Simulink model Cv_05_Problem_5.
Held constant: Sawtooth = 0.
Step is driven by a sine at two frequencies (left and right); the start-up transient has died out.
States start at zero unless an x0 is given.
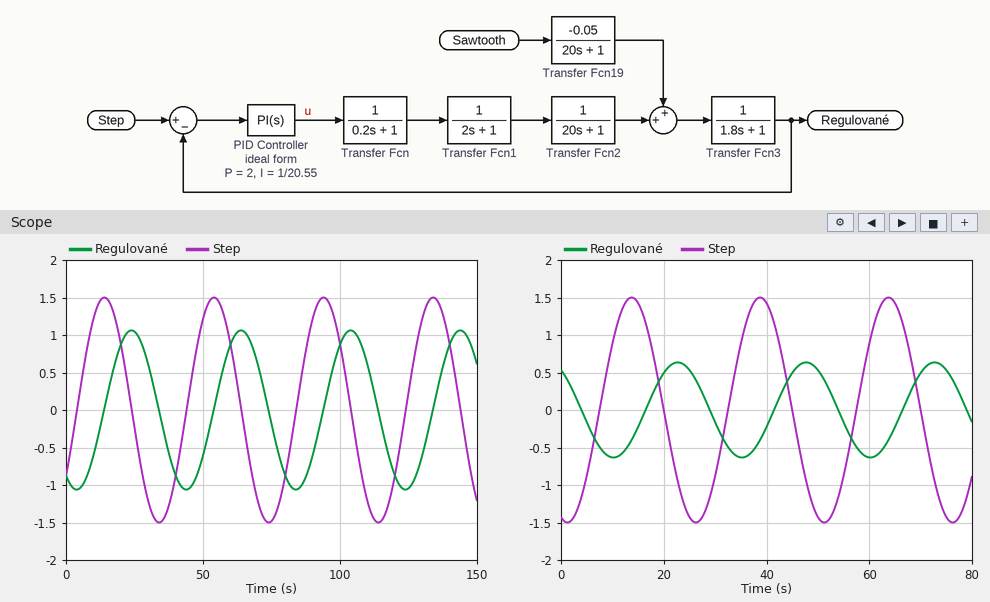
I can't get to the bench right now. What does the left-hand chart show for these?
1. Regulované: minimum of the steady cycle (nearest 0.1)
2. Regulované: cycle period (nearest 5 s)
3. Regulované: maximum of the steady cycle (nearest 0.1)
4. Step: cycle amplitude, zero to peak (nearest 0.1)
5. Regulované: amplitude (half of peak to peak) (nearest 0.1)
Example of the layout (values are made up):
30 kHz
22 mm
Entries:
-1.1
40 s
1.1
1.5
1.1
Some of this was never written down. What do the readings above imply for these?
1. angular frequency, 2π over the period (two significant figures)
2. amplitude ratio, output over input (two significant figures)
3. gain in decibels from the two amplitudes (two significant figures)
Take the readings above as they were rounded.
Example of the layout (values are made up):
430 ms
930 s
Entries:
0.16 rad/s
0.73
-2.7 dB
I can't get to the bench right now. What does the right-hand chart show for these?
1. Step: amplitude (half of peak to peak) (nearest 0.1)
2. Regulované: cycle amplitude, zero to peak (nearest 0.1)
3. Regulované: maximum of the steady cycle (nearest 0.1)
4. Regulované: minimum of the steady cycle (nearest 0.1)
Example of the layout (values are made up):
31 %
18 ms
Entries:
1.5
0.6
0.6
-0.6
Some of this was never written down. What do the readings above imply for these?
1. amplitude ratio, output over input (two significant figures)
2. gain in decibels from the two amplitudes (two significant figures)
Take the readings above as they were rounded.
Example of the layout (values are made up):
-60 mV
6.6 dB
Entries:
0.40
-8.0 dB
